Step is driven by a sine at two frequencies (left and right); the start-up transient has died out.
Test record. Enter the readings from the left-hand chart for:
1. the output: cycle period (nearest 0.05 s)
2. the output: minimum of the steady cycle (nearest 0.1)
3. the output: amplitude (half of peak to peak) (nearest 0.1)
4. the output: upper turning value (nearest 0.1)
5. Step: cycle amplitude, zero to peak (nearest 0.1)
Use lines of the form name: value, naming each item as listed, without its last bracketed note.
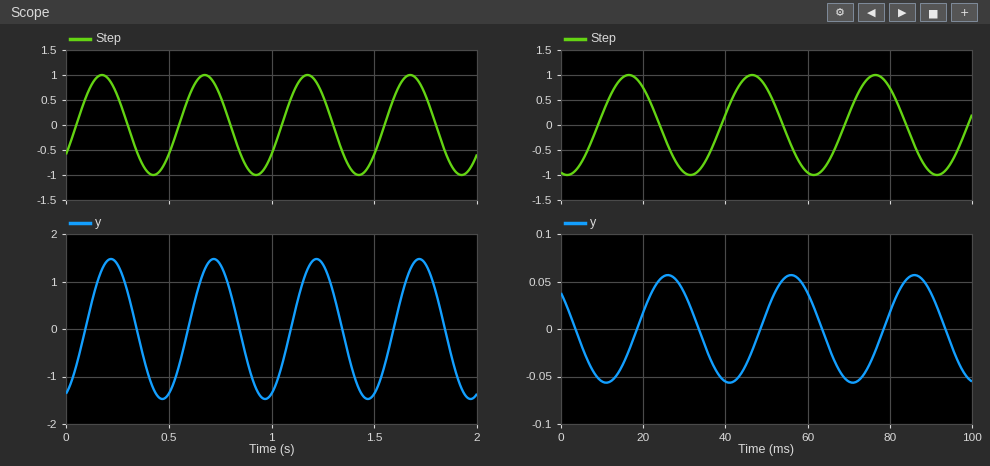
the output: cycle period: 0.50 s
the output: minimum of the steady cycle: -1.5
the output: amplitude (half of peak to peak): 1.5
the output: upper turning value: 1.5
Step: cycle amplitude, zero to peak: 1.0
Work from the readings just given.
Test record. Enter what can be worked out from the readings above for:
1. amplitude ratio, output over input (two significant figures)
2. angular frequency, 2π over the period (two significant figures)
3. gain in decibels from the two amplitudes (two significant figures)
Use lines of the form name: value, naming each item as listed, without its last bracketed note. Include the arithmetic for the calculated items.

amplitude ratio, output over input: 1.5 / 1 = 1.5
angular frequency, 2π over the period: 2π / 0.5 = 13 rad/s
gain in decibels from the two amplitudes: 20 log10(1.5 / 1) = 3.5 dB
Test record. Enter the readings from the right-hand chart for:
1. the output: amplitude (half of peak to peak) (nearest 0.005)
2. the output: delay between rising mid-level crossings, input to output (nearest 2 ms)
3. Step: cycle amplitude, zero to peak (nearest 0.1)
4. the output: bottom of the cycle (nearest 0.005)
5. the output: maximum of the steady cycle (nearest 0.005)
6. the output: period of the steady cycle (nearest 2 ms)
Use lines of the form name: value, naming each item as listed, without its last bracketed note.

the output: amplitude (half of peak to peak): 0.055
the output: delay between rising mid-level crossings, input to output: 10 ms
Step: cycle amplitude, zero to peak: 1.0
the output: bottom of the cycle: -0.055
the output: maximum of the steady cycle: 0.055
the output: period of the steady cycle: 30 ms
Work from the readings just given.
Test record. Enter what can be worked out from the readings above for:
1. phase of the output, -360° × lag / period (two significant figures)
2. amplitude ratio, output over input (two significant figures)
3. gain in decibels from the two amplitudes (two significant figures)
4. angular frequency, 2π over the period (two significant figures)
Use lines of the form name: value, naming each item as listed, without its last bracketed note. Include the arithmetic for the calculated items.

phase of the output, -360° × lag / period: -360 × 10 / 30 = -120°
amplitude ratio, output over input: 0.055 / 1 = 0.055
gain in decibels from the two amplitudes: 20 log10(0.055 / 1) = -25 dB
angular frequency, 2π over the period: 2π / 30 = 0.21 rad/ms
